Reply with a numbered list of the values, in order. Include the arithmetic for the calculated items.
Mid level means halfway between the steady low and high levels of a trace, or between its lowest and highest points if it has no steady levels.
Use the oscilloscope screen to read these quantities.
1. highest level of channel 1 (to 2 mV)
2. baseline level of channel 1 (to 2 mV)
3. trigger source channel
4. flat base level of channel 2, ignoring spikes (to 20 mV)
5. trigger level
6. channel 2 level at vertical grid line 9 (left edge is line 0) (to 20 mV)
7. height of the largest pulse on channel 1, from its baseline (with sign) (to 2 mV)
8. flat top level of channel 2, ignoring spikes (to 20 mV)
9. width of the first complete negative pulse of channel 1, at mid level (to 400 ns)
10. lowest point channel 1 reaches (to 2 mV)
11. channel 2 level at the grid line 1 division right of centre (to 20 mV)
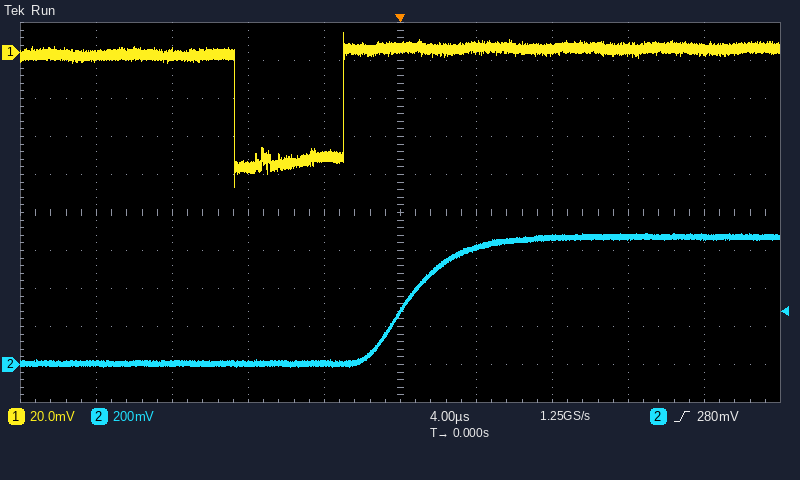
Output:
1. 10 mV
2. 2 mV
3. channel 2
4. 0 mV
5. 280 mV
6. 680 mV
7. -70 mV − (2 mV) = -72 mV
8. 680 mV
9. 5.6 µs
10. -70 mV
11. 620 mV
